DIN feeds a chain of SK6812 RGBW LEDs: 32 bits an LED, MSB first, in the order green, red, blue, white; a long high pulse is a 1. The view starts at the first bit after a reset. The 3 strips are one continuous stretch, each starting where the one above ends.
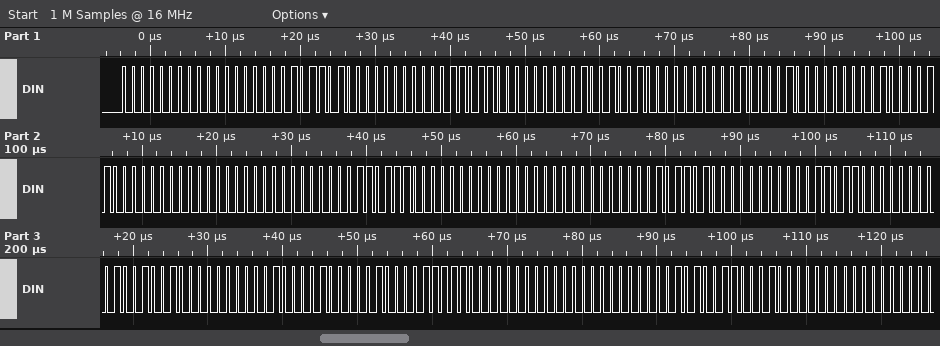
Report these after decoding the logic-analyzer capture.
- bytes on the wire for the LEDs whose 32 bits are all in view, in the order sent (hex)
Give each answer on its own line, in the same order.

00 00 2D 00 1B 00 49 00 21 00 43 00 00 00 37 00 00 00 2D 00 1B 00 49 00 21 04 3E 00 00 05 31 00
